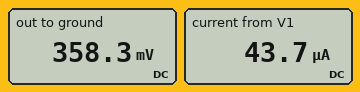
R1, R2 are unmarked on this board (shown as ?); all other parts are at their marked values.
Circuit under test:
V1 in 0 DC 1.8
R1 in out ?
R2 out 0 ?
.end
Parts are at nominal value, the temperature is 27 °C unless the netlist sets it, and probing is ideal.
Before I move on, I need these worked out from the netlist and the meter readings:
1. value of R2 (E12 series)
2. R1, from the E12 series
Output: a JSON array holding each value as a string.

["8.2 kΩ", "33 kΩ"]
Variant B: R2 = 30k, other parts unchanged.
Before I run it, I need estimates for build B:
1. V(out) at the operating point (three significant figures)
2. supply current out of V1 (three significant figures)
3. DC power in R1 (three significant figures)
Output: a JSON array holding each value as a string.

["857 mV", "28.6 µA", "26.9 µW"]
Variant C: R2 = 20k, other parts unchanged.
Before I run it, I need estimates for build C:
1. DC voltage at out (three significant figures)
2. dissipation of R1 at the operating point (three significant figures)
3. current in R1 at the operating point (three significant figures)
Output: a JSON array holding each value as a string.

["679 mV", "38.1 µW", "34.0 µA"]
